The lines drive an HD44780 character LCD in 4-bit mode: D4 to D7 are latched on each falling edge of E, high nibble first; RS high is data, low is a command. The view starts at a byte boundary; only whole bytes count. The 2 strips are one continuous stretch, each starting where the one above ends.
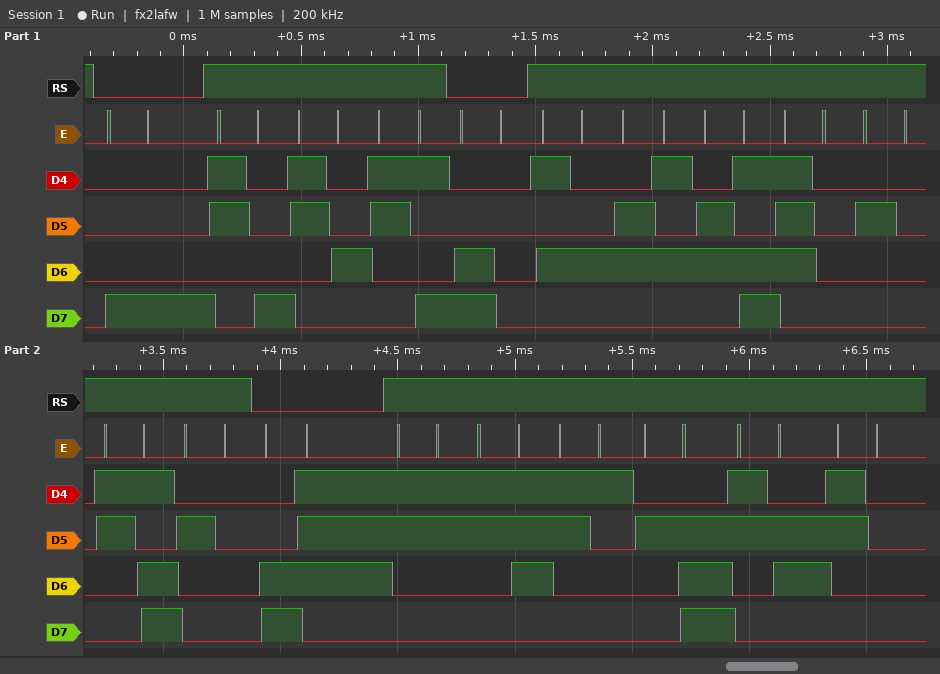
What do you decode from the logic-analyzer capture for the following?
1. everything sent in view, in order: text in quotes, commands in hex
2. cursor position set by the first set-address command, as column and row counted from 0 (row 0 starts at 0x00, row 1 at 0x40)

0x88 "849" 0xC0 "Temp = " 0xC7 "371.60"
column 8, row 0
